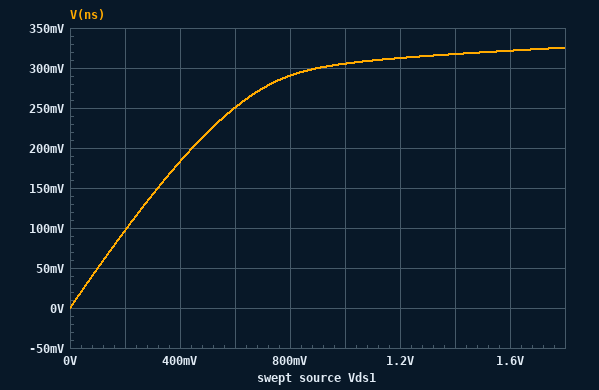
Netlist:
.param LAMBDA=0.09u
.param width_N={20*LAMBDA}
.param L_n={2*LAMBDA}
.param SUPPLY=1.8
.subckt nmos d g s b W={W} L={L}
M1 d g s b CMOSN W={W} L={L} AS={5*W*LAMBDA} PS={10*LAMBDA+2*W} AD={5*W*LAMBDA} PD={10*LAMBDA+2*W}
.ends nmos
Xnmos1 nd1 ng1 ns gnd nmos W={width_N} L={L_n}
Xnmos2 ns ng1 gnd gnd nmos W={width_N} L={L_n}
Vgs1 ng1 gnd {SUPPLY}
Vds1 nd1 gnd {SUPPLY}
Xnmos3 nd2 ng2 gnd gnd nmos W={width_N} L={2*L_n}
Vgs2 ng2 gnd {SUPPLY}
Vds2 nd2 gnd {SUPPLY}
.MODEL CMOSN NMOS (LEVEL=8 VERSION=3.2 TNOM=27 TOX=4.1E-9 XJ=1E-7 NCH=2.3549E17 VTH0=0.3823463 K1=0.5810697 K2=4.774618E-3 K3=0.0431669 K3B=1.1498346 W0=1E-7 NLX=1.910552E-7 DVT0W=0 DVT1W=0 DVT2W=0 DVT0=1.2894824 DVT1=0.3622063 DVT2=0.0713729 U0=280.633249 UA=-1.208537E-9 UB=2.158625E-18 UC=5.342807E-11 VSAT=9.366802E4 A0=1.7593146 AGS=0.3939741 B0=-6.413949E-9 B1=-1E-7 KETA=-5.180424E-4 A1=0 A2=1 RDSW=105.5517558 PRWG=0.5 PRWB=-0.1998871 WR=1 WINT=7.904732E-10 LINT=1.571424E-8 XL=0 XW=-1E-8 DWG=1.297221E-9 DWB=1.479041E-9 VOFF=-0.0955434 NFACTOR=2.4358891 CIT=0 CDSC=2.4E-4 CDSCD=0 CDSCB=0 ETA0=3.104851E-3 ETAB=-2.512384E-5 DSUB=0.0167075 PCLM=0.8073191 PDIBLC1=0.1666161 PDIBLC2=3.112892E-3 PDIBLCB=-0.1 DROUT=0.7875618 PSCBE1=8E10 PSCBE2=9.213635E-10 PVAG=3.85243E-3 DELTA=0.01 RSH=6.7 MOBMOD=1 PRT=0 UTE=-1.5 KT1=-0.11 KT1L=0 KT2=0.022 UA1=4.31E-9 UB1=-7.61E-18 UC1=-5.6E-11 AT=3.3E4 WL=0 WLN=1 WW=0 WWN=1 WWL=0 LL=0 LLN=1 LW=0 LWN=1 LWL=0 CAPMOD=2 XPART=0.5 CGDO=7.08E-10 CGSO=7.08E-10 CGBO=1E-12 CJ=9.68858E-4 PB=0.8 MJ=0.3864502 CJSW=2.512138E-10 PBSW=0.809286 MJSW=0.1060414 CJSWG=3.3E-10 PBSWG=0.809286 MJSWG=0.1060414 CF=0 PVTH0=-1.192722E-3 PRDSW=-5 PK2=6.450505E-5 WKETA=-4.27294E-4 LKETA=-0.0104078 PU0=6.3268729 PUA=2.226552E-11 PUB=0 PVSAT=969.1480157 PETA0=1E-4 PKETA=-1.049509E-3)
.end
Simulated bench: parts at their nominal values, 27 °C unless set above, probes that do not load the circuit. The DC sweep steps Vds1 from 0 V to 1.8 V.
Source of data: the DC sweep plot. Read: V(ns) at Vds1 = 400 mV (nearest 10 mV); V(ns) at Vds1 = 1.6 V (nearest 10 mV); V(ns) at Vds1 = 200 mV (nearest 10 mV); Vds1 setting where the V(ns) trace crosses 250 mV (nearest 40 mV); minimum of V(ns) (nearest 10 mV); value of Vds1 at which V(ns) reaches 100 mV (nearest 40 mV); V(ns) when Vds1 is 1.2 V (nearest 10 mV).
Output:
180 mV
320 mV
100 mV
600 mV
0 V
200 mV
310 mV
